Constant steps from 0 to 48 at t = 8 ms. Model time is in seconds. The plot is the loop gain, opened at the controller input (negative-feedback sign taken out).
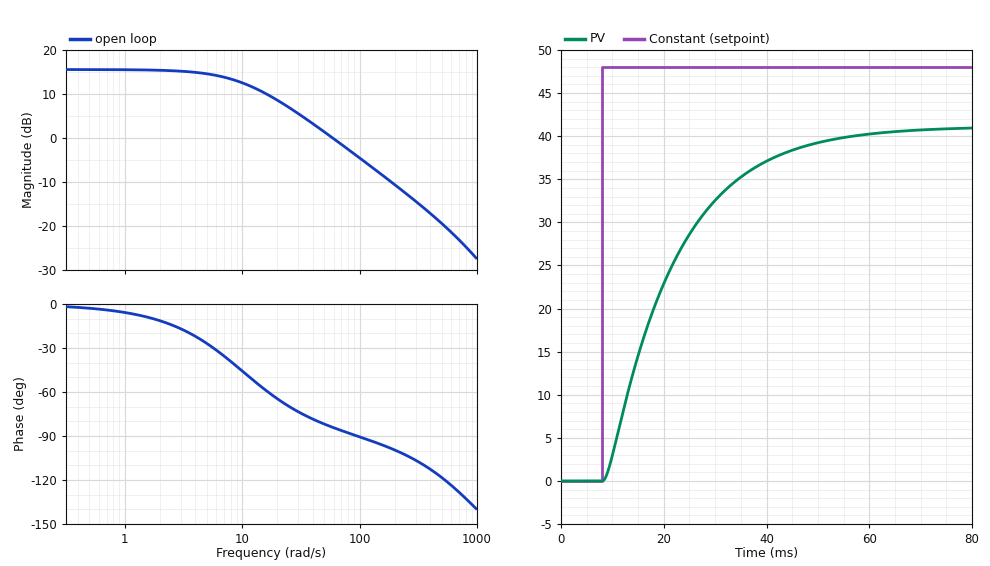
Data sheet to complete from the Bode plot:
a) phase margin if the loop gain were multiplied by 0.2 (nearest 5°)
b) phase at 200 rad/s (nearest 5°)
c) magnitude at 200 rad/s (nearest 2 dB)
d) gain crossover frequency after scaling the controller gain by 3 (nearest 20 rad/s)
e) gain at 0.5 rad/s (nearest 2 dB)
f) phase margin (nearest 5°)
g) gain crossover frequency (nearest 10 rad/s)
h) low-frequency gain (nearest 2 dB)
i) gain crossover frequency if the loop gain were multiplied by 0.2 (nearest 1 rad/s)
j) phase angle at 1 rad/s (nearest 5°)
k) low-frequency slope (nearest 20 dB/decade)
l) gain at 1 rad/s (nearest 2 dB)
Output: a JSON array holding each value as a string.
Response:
["145°", "-100°", "-10 dB", "180 rad/s", "16 dB", "95°", "60 rad/s", "16 dB", "7 rad/s", "-5°", "0 dB/decade", "16 dB"]
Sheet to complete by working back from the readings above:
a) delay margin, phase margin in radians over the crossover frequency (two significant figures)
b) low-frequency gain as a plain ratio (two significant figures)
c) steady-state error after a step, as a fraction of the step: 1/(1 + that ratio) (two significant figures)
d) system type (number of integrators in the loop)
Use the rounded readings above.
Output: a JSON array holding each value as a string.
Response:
["0.028 s", "6.3", "0.14", "0"]
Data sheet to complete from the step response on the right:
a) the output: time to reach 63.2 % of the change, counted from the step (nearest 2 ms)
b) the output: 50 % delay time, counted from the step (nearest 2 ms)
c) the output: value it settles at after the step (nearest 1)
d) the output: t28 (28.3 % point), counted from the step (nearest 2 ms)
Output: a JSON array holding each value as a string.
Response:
["14 ms", "10 ms", "41", "6 ms"]
